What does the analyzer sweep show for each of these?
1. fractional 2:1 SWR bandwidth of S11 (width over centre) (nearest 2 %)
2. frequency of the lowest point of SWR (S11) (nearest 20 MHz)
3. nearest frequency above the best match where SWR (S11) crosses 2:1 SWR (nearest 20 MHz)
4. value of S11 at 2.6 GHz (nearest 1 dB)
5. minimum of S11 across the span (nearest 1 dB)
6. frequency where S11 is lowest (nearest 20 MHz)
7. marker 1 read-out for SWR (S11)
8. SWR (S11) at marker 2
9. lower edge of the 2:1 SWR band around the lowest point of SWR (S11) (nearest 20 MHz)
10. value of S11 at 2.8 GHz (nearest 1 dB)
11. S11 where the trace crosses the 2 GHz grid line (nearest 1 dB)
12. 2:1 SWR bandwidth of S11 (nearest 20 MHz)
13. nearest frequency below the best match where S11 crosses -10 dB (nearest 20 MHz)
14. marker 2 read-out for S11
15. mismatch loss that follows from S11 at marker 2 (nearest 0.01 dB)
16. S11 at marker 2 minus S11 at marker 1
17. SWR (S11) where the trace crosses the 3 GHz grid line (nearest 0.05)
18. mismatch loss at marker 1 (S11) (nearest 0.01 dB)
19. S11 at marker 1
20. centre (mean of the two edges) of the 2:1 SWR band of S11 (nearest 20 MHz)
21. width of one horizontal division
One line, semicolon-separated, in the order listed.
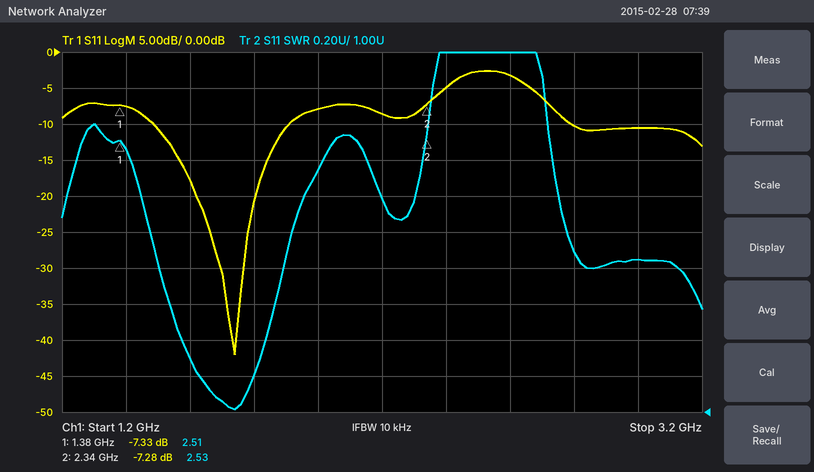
26 %; 1.74 GHz; 1.92 GHz; -3 dB; -42 dB; 1.74 GHz; 2.51; 2.53; 1.48 GHz; -10 dB; -8 dB; 440 MHz; 1.48 GHz; -7.28 dB; 0.90 dB; 0.05 dB; 1.85; 0.89 dB; -7.33 dB; 1.70 GHz; 200 MHz
